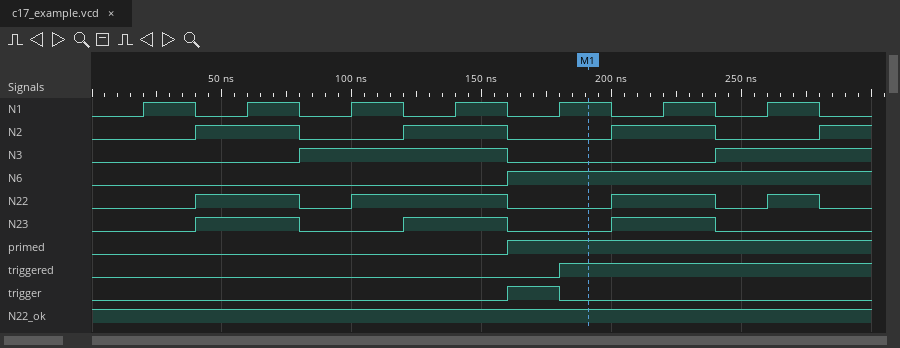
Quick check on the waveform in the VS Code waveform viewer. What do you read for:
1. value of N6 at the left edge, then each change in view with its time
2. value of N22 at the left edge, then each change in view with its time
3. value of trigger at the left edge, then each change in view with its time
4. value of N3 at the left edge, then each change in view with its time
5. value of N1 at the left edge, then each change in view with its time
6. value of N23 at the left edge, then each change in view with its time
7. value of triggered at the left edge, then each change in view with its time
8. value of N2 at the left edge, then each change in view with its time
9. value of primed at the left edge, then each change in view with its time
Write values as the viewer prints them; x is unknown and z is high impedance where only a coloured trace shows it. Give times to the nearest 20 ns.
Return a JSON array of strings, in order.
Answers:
["0, 1 at 160 ns", "0, 1 at 40 ns, 0 at 80 ns, 1 at 100 ns, 0 at 160 ns, 1 at 200 ns, 0 at 240 ns, 1 at 260 ns, 0 at 280 ns", "0, 1 at 160 ns, 0 at 180 ns", "0, 1 at 80 ns, 0 at 160 ns, 1 at 240 ns", "0, 1 at 20 ns, 0 at 40 ns, 1 at 60 ns, 0 at 80 ns, 1 at 100 ns, 0 at 120 ns, 1 at 140 ns, 0 at 160 ns, 1 at 180 ns, 0 at 200 ns, 1 at 220 ns, 0 at 240 ns, 1 at 260 ns, 0 at 280 ns", "0, 1 at 40 ns, 0 at 80 ns, 1 at 120 ns, 0 at 160 ns, 1 at 200 ns, 0 at 240 ns", "0, 1 at 180 ns", "0, 1 at 40 ns, 0 at 80 ns, 1 at 120 ns, 0 at 160 ns, 1 at 200 ns, 0 at 240 ns, 1 at 280 ns", "0, 1 at 160 ns"]
